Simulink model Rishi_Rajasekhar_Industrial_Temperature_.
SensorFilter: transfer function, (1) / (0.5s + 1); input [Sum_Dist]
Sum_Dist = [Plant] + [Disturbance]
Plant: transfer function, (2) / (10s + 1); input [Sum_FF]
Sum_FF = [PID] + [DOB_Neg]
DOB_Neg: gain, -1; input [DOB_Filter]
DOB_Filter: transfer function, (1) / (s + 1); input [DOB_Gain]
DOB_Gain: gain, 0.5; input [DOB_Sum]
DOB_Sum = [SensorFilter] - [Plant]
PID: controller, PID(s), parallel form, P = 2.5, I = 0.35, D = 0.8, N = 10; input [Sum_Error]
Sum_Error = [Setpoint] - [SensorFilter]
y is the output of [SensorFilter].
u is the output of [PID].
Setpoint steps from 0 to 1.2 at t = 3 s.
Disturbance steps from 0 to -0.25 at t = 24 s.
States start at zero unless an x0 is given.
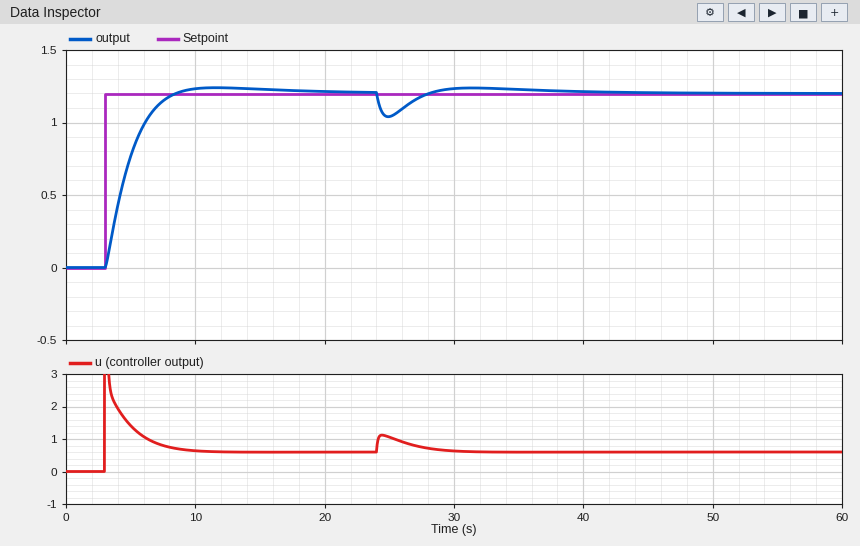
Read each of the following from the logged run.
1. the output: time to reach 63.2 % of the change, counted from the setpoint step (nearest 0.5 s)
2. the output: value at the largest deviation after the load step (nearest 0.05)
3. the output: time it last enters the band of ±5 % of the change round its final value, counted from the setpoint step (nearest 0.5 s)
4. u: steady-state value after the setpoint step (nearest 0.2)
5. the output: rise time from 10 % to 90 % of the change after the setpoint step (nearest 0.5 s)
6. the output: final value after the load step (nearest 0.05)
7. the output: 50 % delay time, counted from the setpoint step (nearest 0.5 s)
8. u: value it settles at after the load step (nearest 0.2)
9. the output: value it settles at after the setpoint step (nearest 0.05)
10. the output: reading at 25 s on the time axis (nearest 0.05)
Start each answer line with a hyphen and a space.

- 2.0 s
- 1.05
- 4.5 s
- 0.6
- 3.5 s
- 1.20
- 1.5 s
- 0.6
- 1.20
- 1.05
